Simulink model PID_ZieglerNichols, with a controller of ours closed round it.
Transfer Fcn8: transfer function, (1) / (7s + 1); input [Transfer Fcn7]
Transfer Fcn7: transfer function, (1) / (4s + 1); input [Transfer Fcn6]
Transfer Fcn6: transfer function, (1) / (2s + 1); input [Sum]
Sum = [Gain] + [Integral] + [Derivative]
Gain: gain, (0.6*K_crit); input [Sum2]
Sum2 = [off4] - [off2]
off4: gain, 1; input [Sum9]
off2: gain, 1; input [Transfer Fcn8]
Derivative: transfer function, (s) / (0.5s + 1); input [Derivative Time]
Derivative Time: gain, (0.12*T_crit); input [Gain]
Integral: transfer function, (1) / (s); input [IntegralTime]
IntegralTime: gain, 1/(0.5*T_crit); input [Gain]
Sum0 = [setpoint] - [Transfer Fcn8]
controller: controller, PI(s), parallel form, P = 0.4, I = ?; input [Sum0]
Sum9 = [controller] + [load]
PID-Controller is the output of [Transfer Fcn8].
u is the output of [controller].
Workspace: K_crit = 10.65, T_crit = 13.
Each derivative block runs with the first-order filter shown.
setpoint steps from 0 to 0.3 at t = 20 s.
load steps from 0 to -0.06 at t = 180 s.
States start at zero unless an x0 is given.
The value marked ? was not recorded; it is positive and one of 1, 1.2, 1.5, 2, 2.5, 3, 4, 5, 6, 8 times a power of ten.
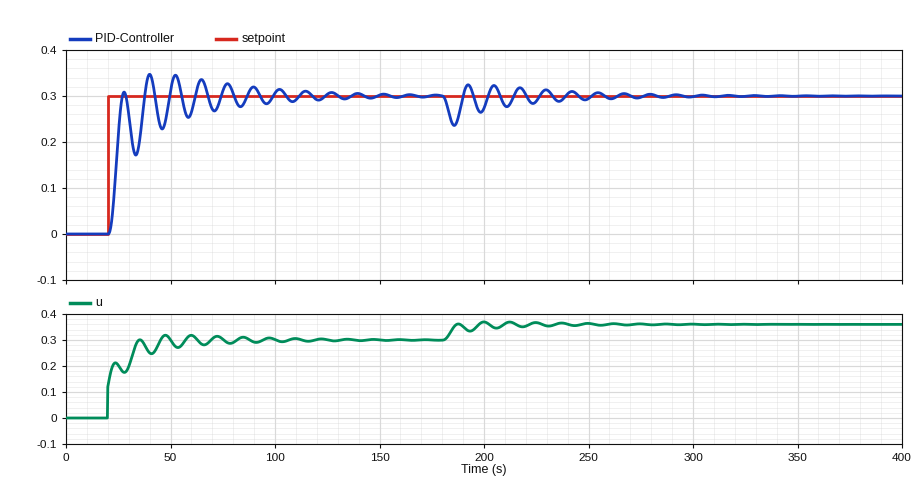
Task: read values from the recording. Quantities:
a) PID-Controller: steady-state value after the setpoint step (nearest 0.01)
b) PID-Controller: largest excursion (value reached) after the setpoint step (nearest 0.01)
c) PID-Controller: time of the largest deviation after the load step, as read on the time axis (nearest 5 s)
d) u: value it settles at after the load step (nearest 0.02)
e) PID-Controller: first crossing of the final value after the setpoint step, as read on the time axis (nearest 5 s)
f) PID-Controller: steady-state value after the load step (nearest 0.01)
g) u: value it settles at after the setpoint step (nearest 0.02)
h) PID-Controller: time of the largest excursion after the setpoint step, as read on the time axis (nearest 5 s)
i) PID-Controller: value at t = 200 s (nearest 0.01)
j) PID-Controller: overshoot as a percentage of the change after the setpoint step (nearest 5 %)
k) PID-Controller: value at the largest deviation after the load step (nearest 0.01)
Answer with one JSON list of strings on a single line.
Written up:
["0.30", "0.35", "185 s", "0.36", "25 s", "0.30", "0.30", "40 s", "0.27", "15 %", "0.24"]
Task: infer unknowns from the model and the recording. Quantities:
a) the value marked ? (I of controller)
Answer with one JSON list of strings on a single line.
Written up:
["0.15"]
